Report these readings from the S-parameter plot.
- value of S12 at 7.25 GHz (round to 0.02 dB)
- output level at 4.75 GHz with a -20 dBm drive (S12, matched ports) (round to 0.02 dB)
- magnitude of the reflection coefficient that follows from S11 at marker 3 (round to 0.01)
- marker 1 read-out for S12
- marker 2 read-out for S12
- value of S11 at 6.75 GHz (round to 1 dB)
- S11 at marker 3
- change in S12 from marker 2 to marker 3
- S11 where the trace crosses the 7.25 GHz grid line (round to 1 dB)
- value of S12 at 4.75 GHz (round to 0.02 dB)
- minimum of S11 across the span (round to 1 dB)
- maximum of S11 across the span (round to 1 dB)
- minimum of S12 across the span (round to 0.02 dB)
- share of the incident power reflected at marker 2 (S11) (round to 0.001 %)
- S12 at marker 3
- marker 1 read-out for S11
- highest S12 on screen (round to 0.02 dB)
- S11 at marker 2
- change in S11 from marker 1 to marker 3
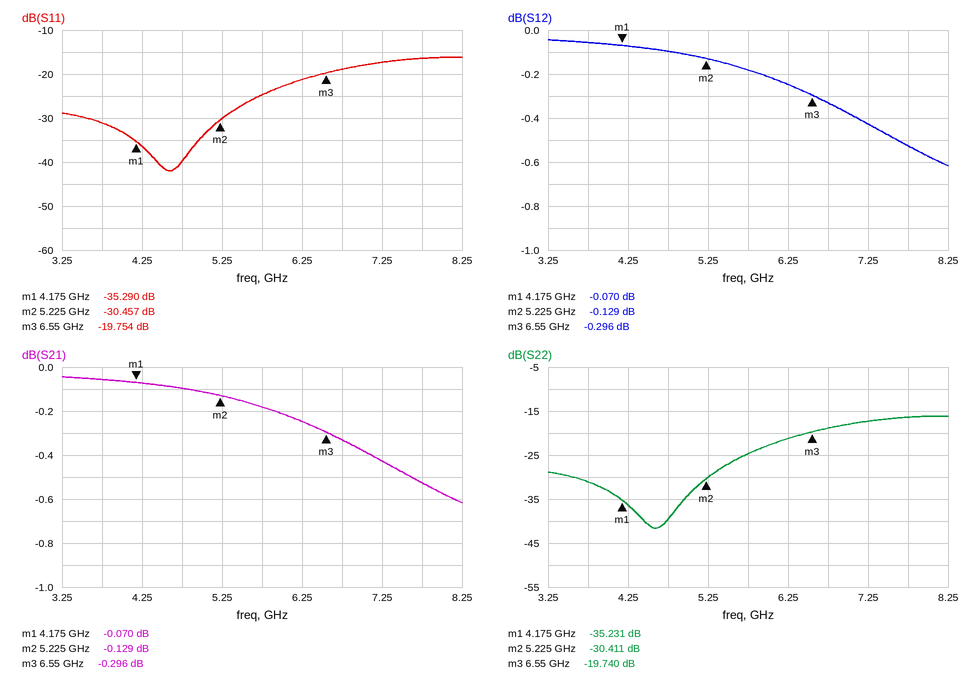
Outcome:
-0.42 dB
-20.10 dBm
0.10
-0.070 dB
-0.129 dB
-19 dB
-19.754 dB
-0.167 dB
-17 dB
-0.10 dB
-42 dB
-16 dB
-0.62 dB
0.090 %
-0.296 dB
-35.290 dB
-0.04 dB
-30.457 dB
15.536 dB
